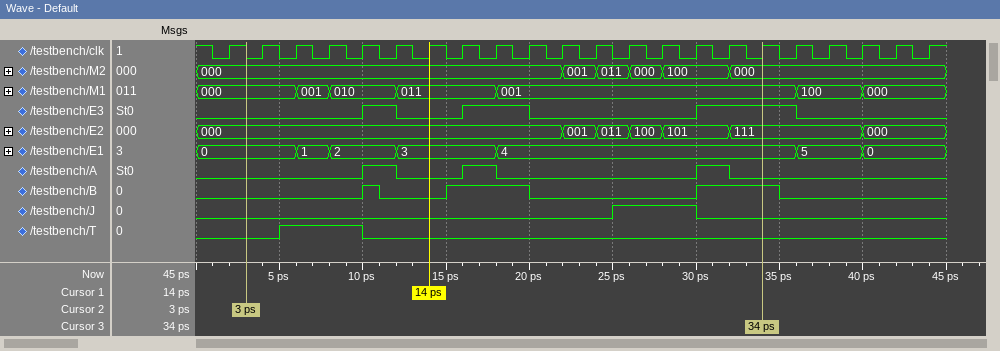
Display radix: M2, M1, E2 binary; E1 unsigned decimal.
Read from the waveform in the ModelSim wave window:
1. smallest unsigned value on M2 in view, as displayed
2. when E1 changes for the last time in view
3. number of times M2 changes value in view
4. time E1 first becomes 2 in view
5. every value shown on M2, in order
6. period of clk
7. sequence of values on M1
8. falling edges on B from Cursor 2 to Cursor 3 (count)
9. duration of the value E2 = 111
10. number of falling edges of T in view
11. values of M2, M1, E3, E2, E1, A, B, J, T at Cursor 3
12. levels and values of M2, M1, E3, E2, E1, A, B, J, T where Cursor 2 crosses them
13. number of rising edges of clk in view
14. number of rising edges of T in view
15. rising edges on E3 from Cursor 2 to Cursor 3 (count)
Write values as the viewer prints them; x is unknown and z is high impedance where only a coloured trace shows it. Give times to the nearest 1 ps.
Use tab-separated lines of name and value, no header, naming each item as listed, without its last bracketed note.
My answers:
smallest unsigned value on M2 in view, as displayed	000
when E1 changes for the last time in view	40 ps
number of times M2 changes value in view	5
time E1 first becomes 2 in view	8 ps
every value shown on M2, in order	000, 001, 011, 000, 100, 000
period of clk	2 ps
sequence of values on M1	000, 001, 010, 011, 001, 100, 000
falling edges on B from Cursor 2 to Cursor 3	2
duration of the value E2 = 111	8 ps
number of falling edges of T in view	1
values of M2, M1, E3, E2, E1, A, B, J, T at Cursor 3	M2=000, M1=001, E3=1, E2=111, E1=4, A=0, B=1, J=0, T=0
levels and values of M2, M1, E3, E2, E1, A, B, J, T where Cursor 2 crosses them	M2=000, M1=000, E3=0, E2=000, E1=0, A=0, B=0, J=0, T=0
number of rising edges of clk in view	22
number of rising edges of T in view	1
rising edges on E3 from Cursor 2 to Cursor 3	3
